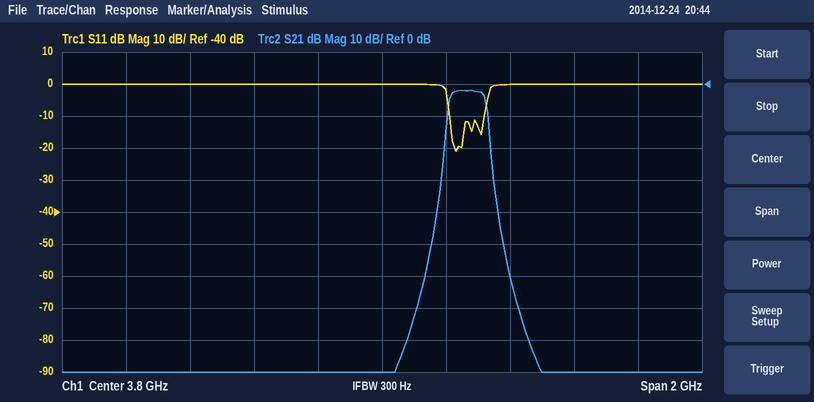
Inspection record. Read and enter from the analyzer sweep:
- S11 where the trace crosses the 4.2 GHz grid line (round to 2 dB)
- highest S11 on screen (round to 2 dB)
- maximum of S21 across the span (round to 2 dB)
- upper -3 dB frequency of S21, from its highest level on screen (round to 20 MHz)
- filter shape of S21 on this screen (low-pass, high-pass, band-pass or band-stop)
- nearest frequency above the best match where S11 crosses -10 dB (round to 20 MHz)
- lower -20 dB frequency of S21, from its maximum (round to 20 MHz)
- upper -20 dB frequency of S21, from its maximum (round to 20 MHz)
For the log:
0 dB
0 dB
-2 dB
4.12 GHz
band-pass
4.12 GHz
4.00 GHz
4.14 GHz
